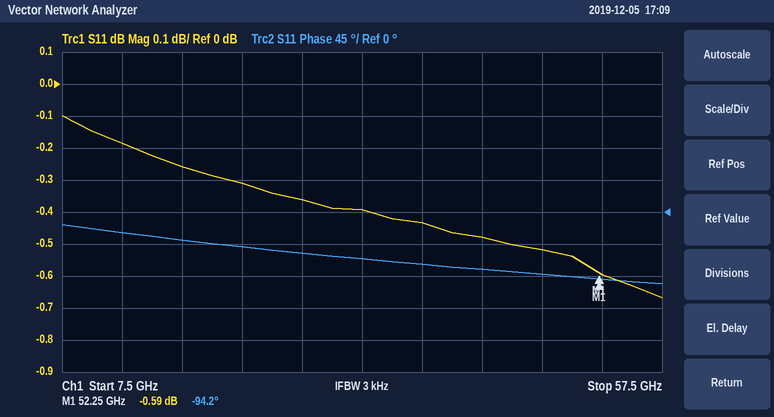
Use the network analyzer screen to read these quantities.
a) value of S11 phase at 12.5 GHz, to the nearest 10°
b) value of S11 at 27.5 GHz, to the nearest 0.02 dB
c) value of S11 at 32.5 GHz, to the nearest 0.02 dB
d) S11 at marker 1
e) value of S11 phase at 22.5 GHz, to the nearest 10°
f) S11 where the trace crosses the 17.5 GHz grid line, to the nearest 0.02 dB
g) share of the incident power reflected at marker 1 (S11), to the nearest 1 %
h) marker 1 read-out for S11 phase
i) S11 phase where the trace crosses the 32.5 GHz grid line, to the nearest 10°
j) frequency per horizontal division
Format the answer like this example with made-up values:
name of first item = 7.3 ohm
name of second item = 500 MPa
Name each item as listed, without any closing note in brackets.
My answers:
value of S11 phase at 12.5 GHz, to the nearest 10° = -30°
value of S11 at 27.5 GHz, to the nearest 0.02 dB = -0.36 dB
value of S11 at 32.5 GHz, to the nearest 0.02 dB = -0.40 dB
S11 at marker 1 = -0.59 dB
value of S11 phase at 22.5 GHz, to the nearest 10° = -50°
S11 where the trace crosses the 17.5 GHz grid line, to the nearest 0.02 dB = -0.26 dB
share of the incident power reflected at marker 1 (S11), to the nearest 1 % = 87 %
marker 1 read-out for S11 phase = -94.2°
S11 phase where the trace crosses the 32.5 GHz grid line, to the nearest 10° = -70°
frequency per horizontal division = 5 GHz
